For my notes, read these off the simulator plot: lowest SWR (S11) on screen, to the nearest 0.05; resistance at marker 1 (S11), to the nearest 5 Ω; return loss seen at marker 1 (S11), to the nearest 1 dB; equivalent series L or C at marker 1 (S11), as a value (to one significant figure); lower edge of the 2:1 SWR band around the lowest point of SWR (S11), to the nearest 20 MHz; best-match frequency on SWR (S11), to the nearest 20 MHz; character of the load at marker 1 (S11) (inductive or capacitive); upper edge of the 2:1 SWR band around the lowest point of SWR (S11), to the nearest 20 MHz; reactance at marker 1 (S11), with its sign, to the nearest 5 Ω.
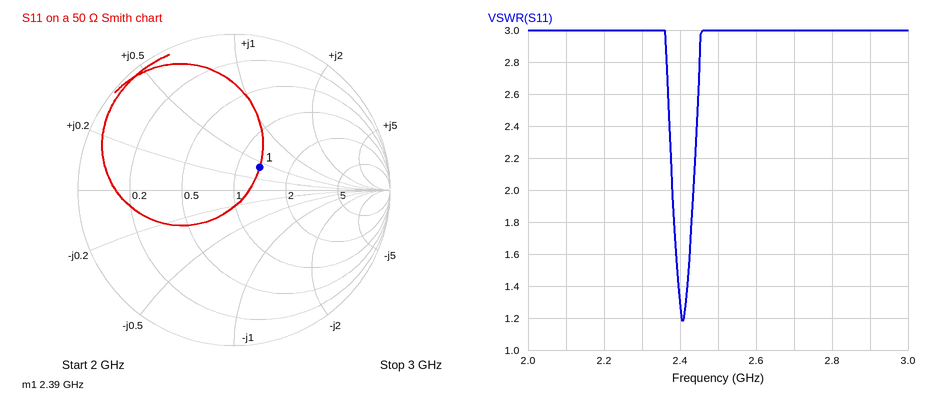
1.20
65 Ω
13 dB
1 nH
2.38 GHz
2.40 GHz
inductive
2.44 GHz
+20 Ω
